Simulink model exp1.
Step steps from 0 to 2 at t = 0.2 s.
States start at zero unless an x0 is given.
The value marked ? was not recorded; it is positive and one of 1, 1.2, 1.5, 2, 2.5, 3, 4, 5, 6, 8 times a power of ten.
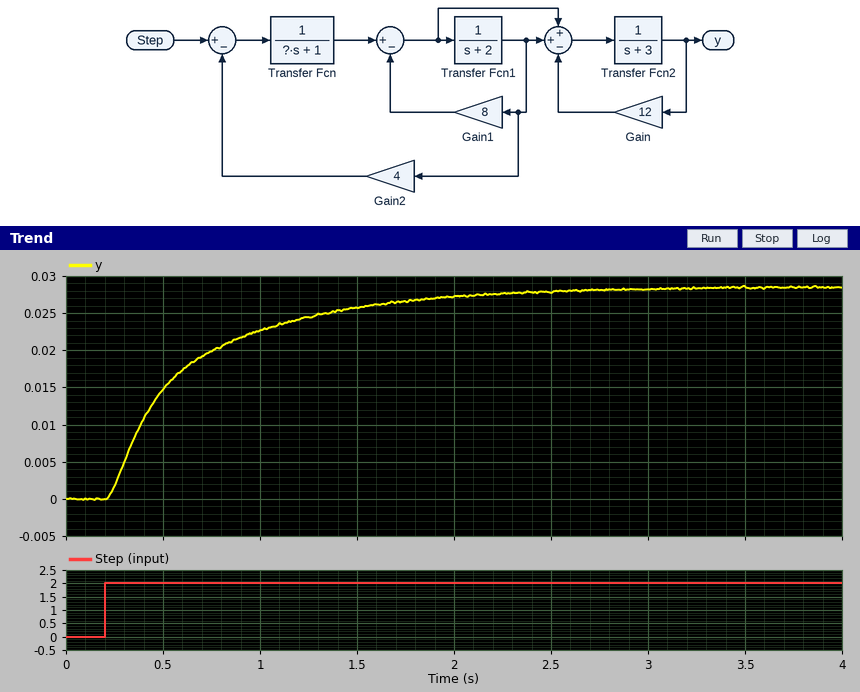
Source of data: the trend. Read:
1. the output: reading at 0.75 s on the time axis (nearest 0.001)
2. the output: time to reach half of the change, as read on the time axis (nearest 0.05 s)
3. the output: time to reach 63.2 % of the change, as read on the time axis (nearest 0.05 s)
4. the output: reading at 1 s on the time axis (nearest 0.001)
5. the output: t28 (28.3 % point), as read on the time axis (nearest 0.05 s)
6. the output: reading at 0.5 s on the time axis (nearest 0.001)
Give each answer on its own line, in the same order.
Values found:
0.020
0.50 s
0.65 s
0.023
0.35 s
0.015
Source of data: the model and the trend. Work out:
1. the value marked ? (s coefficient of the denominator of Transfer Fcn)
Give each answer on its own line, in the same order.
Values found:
1
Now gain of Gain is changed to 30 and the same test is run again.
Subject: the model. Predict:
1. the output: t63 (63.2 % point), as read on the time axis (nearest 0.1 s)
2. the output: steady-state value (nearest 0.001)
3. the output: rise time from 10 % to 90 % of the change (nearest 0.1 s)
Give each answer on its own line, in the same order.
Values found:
0.6 s
0.013
1.2 s
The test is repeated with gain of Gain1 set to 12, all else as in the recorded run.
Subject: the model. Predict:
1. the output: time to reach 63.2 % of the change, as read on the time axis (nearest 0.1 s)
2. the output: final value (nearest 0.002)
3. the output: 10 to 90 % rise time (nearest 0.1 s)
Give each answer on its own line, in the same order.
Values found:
0.7 s
0.022
1.4 s
